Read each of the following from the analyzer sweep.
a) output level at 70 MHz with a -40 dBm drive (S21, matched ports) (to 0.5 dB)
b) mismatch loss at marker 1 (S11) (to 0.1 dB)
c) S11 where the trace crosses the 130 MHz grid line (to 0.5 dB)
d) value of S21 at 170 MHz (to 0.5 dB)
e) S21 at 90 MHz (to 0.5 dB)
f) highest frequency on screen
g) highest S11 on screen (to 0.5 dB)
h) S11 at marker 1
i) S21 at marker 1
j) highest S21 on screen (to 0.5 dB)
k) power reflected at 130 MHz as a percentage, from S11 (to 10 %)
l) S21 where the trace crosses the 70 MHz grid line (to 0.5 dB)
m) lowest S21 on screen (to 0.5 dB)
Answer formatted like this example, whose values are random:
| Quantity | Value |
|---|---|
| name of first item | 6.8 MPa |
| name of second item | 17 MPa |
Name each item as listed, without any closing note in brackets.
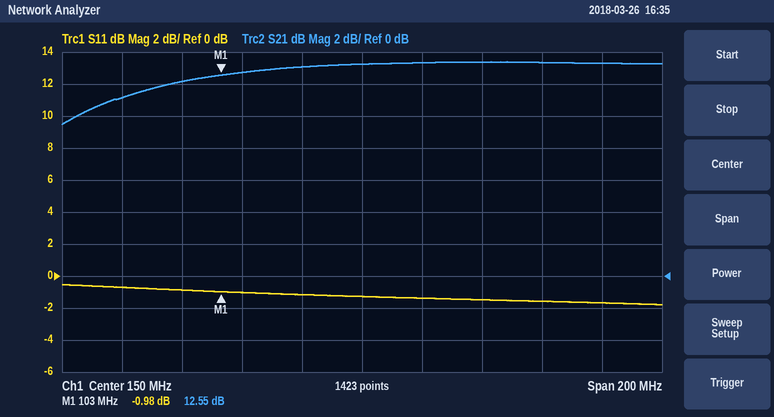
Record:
| Quantity | Value |
|---|---|
| output level at 70 MHz with a -40 dBm drive (S21, matched ports) | -29.0 dBm |
| mismatch loss at marker 1 (S11) | 6.9 dB |
| S11 where the trace crosses the 130 MHz grid line | -1.0 dB |
| value of S21 at 170 MHz | 13.5 dB |
| S21 at 90 MHz | 12.0 dB |
| highest frequency on screen | 250 MHz |
| highest S11 on screen | -0.5 dB |
| S11 at marker 1 | -0.98 dB |
| S21 at marker 1 | 12.55 dB |
| highest S21 on screen | 13.5 dB |
| power reflected at 130 MHz as a percentage, from S11 | 80 % |
| S21 where the trace crosses the 70 MHz grid line | 11.0 dB |
| lowest S21 on screen | 9.5 dB |
